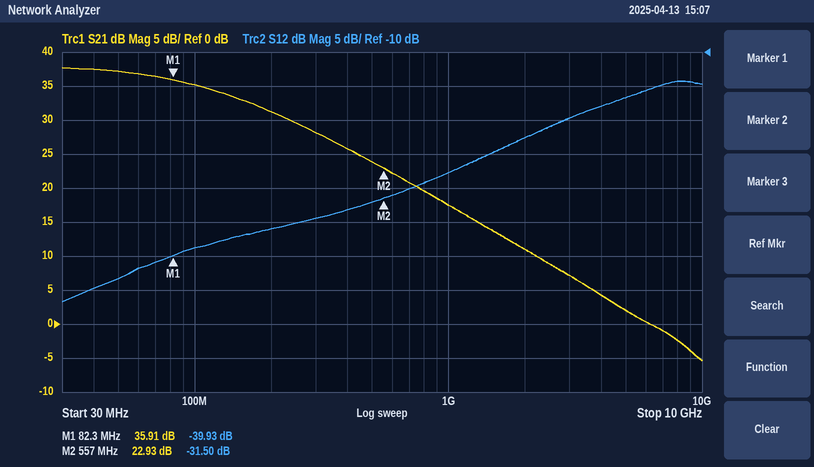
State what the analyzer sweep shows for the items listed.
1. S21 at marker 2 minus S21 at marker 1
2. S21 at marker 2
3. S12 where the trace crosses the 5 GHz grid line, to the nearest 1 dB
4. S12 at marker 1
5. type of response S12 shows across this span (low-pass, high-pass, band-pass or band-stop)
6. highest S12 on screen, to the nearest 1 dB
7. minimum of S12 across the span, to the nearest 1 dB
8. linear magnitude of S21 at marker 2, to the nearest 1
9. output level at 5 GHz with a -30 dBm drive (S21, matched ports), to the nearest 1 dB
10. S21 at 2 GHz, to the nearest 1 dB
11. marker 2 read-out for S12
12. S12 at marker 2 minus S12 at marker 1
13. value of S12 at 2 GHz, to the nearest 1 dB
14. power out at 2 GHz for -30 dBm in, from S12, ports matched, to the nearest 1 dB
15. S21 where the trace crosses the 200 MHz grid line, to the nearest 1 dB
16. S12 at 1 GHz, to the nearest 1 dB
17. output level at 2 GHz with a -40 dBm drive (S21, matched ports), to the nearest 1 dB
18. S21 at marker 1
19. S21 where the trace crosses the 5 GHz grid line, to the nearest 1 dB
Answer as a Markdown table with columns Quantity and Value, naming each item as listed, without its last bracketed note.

| Quantity | Value |
|---|---|
| S21 at marker 2 minus S21 at marker 1 | -12.98 dB |
| S21 at marker 2 | 22.93 dB |
| S12 where the trace crosses the 5 GHz grid line, to the nearest 1 dB | -17 dB |
| S12 at marker 1 | -39.93 dB |
| type of response S12 shows across this span | high-pass |
| highest S12 on screen, to the nearest 1 dB | -14 dB |
| minimum of S12 across the span, to the nearest 1 dB | -47 dB |
| linear magnitude of S21 at marker 2, to the nearest 1 | 14 |
| output level at 5 GHz with a -30 dBm drive (S21, matched ports), to the nearest 1 dB | -28 dBm |
| S21 at 2 GHz, to the nearest 1 dB | 11 dB |
| marker 2 read-out for S12 | -31.50 dB |
| S12 at marker 2 minus S12 at marker 1 | 8.43 dB |
| value of S12 at 2 GHz, to the nearest 1 dB | -23 dB |
| power out at 2 GHz for -30 dBm in, from S12, ports matched, to the nearest 1 dB | -53 dBm |
| S21 where the trace crosses the 200 MHz grid line, to the nearest 1 dB | 31 dB |
| S12 at 1 GHz, to the nearest 1 dB | -28 dB |
| output level at 2 GHz with a -40 dBm drive (S21, matched ports), to the nearest 1 dB | -29 dBm |
| S21 at marker 1 | 35.91 dB |
| S21 where the trace crosses the 5 GHz grid line, to the nearest 1 dB | 2 dB |
